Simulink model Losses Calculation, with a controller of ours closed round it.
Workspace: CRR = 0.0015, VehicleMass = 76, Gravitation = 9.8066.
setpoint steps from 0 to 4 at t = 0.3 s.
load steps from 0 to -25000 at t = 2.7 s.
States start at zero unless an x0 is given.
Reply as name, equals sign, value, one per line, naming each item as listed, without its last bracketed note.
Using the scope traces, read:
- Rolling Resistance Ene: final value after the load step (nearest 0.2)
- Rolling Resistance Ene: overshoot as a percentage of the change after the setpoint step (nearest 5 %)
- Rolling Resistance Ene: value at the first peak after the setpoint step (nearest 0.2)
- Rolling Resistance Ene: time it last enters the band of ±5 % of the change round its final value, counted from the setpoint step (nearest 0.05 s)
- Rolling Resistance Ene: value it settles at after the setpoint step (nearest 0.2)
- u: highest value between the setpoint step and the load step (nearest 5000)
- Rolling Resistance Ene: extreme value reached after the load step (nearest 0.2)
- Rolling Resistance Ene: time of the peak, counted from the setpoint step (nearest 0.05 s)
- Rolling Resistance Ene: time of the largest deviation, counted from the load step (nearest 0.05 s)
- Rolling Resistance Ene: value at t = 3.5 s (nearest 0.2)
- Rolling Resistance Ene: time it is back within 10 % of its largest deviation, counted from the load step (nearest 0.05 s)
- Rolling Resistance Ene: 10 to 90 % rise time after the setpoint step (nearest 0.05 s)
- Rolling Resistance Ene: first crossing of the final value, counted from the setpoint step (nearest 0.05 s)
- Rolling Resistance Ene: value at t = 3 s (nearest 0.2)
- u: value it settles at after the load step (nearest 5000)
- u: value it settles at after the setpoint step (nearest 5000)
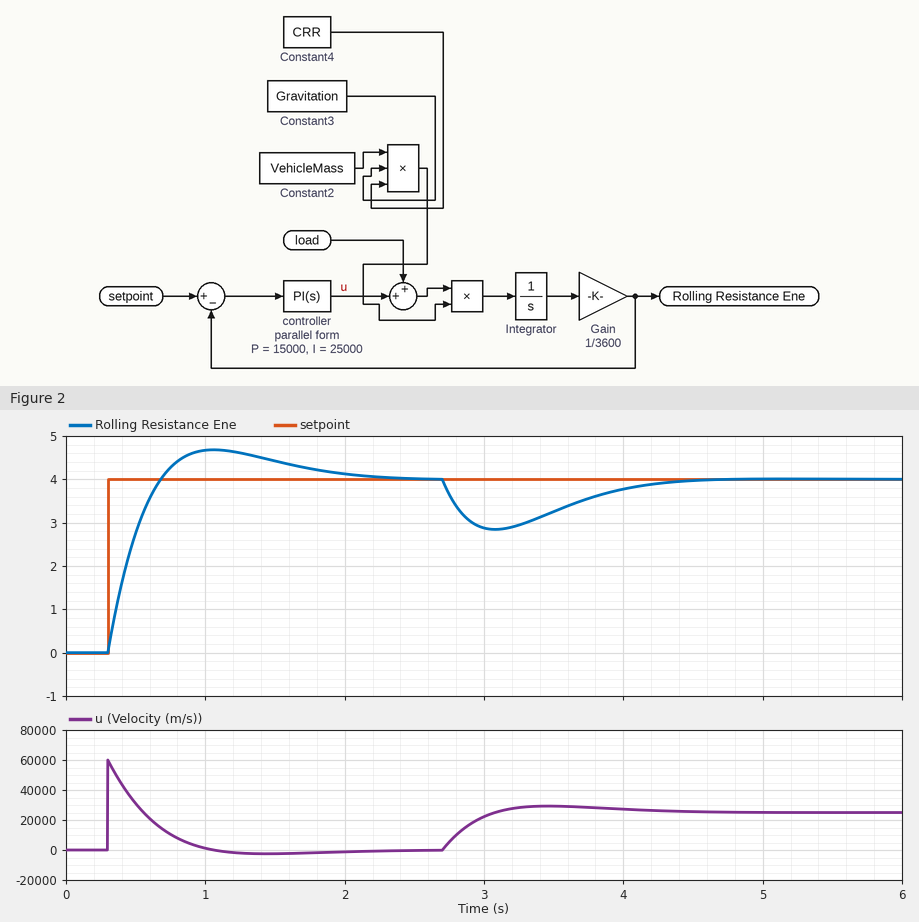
Rolling Resistance Ene: final value after the load step = 4.0
Rolling Resistance Ene: overshoot as a percentage of the change after the setpoint step = 15 %
Rolling Resistance Ene: value at the first peak after the setpoint step = 4.6
Rolling Resistance Ene: time it last enters the band of ±5 % of the change round its final value, counted from the setpoint step = 1.55 s
Rolling Resistance Ene: value it settles at after the setpoint step = 4.0
u: highest value between the setpoint step and the load step = 60000
Rolling Resistance Ene: extreme value reached after the load step = 2.8
Rolling Resistance Ene: time of the peak, counted from the setpoint step = 0.75 s
Rolling Resistance Ene: time of the largest deviation, counted from the load step = 0.40 s
Rolling Resistance Ene: value at t = 3.5 s = 3.2
Rolling Resistance Ene: time it is back within 10 % of its largest deviation, counted from the load step = 1.50 s
Rolling Resistance Ene: 10 to 90 % rise time after the setpoint step = 0.30 s
Rolling Resistance Ene: first crossing of the final value, counted from the setpoint step = 0.40 s
Rolling Resistance Ene: value at t = 3 s = 2.8
u: value it settles at after the load step = 25000
u: value it settles at after the setpoint step = 0
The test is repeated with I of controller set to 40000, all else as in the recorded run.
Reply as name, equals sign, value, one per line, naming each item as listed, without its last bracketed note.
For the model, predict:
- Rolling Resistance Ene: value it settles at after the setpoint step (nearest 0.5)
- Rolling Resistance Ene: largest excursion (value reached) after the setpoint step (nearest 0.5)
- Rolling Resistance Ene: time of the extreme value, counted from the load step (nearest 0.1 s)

Rolling Resistance Ene: value it settles at after the setpoint step = 4.0
Rolling Resistance Ene: largest excursion (value reached) after the setpoint step = 5.0
Rolling Resistance Ene: time of the extreme value, counted from the load step = 0.3 s
